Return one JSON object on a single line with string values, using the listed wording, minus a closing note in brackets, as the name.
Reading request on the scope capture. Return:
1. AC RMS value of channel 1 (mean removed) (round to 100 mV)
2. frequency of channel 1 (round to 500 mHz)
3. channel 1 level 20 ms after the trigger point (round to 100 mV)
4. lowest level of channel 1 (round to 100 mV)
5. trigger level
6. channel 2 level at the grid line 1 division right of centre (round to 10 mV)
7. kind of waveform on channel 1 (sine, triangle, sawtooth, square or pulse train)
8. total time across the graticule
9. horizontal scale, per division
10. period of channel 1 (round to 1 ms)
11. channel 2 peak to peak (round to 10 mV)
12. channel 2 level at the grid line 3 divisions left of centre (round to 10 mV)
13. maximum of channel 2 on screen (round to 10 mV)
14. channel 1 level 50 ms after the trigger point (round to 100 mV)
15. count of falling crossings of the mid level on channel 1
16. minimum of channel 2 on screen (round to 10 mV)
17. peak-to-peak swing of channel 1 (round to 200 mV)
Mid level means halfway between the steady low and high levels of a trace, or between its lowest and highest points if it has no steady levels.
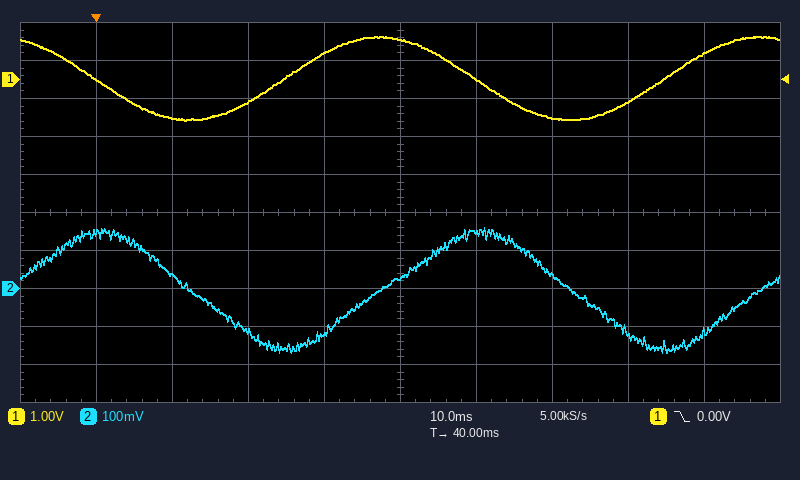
{"AC RMS value of channel 1 (mean removed)": "800 mV", "frequency of channel 1": "20.0 Hz", "channel 1 level 20 ms after the trigger point": "-600 mV", "lowest level of channel 1": "-1.1 V", "trigger level": "0.00 V", "channel 2 level at the grid line 1 division right of centre": "150 mV", "kind of waveform on channel 1": "sine", "total time across the graticule": "100 ms", "horizontal scale, per division": "10 ms", "period of channel 1": "50 ms", "channel 2 peak to peak": "330 mV", "channel 2 level at the grid line 3 divisions left of centre": "40 mV", "maximum of channel 2 on screen": "160 mV", "channel 1 level 50 ms after the trigger point": "0.0 V", "count of falling crossings of the mid level on channel 1": "2", "minimum of channel 2 on screen": "-170 mV", "peak-to-peak swing of channel 1": "2.2 V"}
